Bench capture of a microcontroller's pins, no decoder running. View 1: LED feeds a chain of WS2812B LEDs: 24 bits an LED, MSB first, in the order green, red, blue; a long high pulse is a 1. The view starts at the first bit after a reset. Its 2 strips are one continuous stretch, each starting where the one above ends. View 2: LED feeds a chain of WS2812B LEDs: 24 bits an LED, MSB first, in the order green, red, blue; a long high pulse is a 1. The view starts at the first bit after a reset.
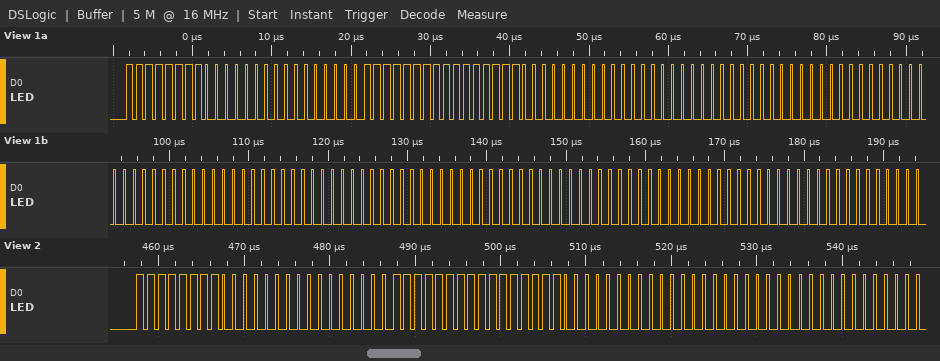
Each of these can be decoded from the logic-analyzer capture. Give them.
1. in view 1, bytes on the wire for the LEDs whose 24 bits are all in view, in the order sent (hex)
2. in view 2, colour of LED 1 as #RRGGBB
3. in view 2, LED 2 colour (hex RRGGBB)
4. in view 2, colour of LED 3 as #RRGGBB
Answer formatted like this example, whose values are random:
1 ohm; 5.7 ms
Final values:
FF 00 00 FF FF 00 00 00 00 00 00 00 00 00 00 00 00 00; #00FF00; #FFFF00; #000000
